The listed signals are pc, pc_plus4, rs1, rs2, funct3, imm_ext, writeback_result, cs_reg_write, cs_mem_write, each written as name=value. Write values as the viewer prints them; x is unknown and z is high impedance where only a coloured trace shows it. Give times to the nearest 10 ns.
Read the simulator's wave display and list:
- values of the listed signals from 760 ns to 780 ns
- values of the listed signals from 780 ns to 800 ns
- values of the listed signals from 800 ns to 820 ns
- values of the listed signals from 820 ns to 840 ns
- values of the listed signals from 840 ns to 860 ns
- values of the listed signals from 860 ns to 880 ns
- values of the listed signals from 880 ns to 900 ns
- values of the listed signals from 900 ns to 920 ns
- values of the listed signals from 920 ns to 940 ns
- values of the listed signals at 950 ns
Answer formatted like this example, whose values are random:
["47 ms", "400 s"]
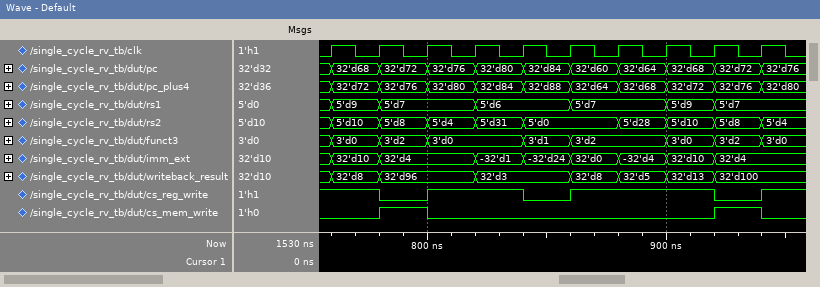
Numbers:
["pc=32'd68, pc_plus4=32'd72, rs1=5'd9, rs2=5'd10, funct3=3'd0, imm_ext=32'd10, writeback_result=32'd8, cs_reg_write=1, cs_mem_write=0", "pc=32'd72, pc_plus4=32'd76, rs1=5'd7, rs2=5'd8, funct3=3'd2, imm_ext=32'd4, writeback_result=32'd96, cs_reg_write=0, cs_mem_write=1", "pc=32'd76, pc_plus4=32'd80, rs1=5'd7, rs2=5'd4, funct3=3'd0, imm_ext=32'd4, writeback_result=32'd96, cs_reg_write=1, cs_mem_write=0", "pc=32'd80, pc_plus4=32'd84, rs1=5'd6, rs2=5'd31, funct3=3'd0, imm_ext=-32'd1, writeback_result=32'd3, cs_reg_write=1, cs_mem_write=0", "pc=32'd84, pc_plus4=32'd88, rs1=5'd6, rs2=5'd0, funct3=3'd1, imm_ext=-32'd24, writeback_result=32'd3, cs_reg_write=0, cs_mem_write=0", "pc=32'd60, pc_plus4=32'd64, rs1=5'd7, rs2=5'd0, funct3=3'd2, imm_ext=32'd0, writeback_result=32'd8, cs_reg_write=1, cs_mem_write=0", "pc=32'd64, pc_plus4=32'd68, rs1=5'd7, rs2=5'd28, funct3=3'd2, imm_ext=-32'd4, writeback_result=32'd5, cs_reg_write=1, cs_mem_write=0", "pc=32'd68, pc_plus4=32'd72, rs1=5'd9, rs2=5'd10, funct3=3'd0, imm_ext=32'd10, writeback_result=32'd13, cs_reg_write=1, cs_mem_write=0", "pc=32'd72, pc_plus4=32'd76, rs1=5'd7, rs2=5'd8, funct3=3'd2, imm_ext=32'd4, writeback_result=32'd100, cs_reg_write=0, cs_mem_write=1", "pc=32'd76, pc_plus4=32'd80, rs1=5'd7, rs2=5'd4, funct3=3'd0, imm_ext=32'd4, writeback_result=32'd100, cs_reg_write=1, cs_mem_write=0"]
